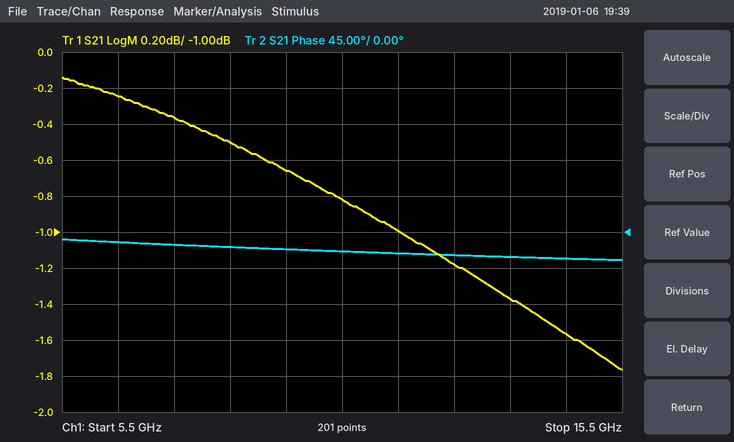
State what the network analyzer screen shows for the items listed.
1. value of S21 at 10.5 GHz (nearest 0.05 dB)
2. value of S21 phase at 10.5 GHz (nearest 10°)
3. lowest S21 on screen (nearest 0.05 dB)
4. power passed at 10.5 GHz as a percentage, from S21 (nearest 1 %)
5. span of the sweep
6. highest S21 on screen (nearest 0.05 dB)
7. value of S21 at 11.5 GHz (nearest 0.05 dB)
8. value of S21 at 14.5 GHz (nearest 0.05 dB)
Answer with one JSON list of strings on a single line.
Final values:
["-0.80 dB", "-20°", "-1.75 dB", "83 %", "10 GHz", "-0.15 dB", "-1.00 dB", "-1.55 dB"]
